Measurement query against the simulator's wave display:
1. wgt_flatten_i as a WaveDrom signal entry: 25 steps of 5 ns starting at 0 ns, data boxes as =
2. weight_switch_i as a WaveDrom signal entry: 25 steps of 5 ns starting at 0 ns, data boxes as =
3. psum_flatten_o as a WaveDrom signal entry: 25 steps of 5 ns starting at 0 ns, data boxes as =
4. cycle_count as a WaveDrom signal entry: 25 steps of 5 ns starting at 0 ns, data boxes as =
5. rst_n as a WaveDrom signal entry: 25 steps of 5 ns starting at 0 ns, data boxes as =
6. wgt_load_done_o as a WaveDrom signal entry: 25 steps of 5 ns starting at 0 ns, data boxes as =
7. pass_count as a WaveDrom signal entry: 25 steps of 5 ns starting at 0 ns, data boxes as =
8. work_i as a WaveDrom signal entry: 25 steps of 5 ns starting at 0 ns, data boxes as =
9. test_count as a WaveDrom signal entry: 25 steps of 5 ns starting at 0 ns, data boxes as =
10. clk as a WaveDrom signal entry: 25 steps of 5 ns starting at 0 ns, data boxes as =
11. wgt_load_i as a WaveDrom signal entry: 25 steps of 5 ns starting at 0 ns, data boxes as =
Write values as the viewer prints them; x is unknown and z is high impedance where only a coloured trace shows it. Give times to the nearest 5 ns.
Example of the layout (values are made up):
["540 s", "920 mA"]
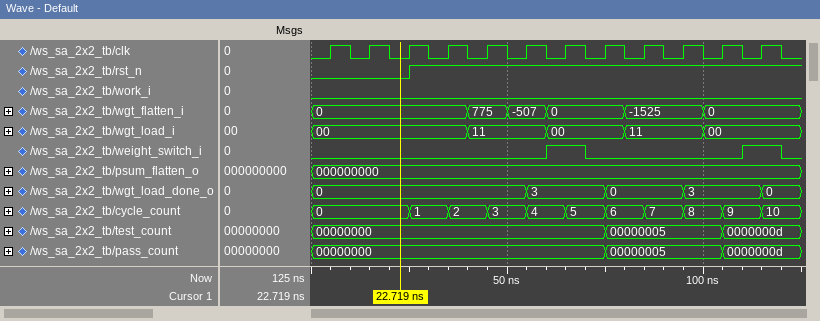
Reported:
["{name: 'wgt_flatten_i', wave: '=.......=.=.=...=...=....', data: '0 775 -507 0 -1525 0'}", "{name: 'weight_switch_i', wave: '0...........1.0.......1.0'}", "{name: 'psum_flatten_o', wave: '=........................', data: '000000000'}", "{name: 'cycle_count', wave: '=....=.=.=.=.=.=.=.=.=.=.', data: '0 1 2 3 4 5 6 7 8 9 10'}", "{name: 'rst_n', wave: '0....1...................'}", "{name: 'wgt_load_done_o', wave: '=..........=...=...=...=.', data: '0 3 0 3 0'}", "{name: 'pass_count', wave: '=..............=.....=...', data: '00000000 00000005 0000000d'}", "{name: 'work_i', wave: '0........................'}", "{name: 'test_count', wave: '=..............=.....=...', data: '00000000 00000005 0000000d'}", "{name: 'clk', wave: '0101010101010101010101010'}", "{name: 'wgt_load_i', wave: '=.......=...=...=...=....', data: '00 11 00 11 00'}"]
